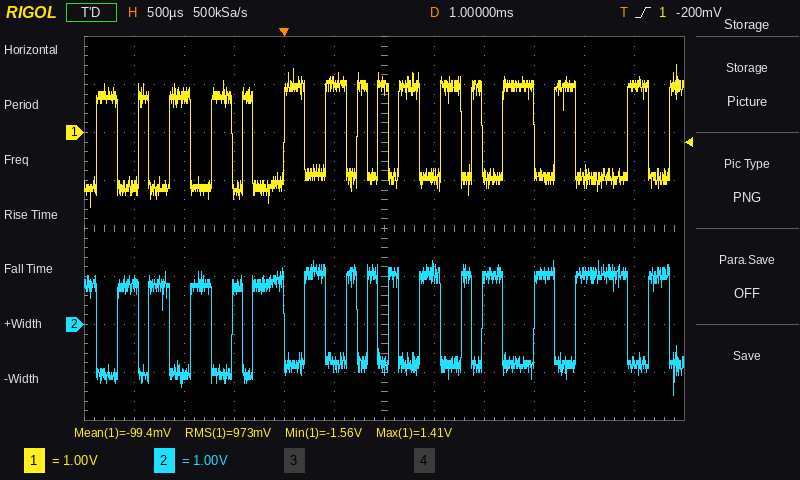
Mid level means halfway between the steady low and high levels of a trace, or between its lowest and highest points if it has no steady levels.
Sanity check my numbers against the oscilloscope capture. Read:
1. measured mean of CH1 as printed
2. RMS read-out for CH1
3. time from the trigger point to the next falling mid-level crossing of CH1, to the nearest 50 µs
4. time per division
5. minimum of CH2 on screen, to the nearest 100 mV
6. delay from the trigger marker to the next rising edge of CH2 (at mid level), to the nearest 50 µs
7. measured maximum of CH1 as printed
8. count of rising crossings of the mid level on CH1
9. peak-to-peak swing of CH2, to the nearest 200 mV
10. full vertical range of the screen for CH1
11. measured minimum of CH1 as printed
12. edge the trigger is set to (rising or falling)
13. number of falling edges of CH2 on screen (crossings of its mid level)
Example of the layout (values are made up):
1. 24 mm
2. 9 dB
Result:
1. -99.4 mV
2. 973 mV
3. 200 µs
4. 500 µs
5. -1.5 V
6. 200 µs
7. 1.41 V
8. 16
9. 2.8 V
10. 8 V
11. -1.56 V
12. rising
13. 16
